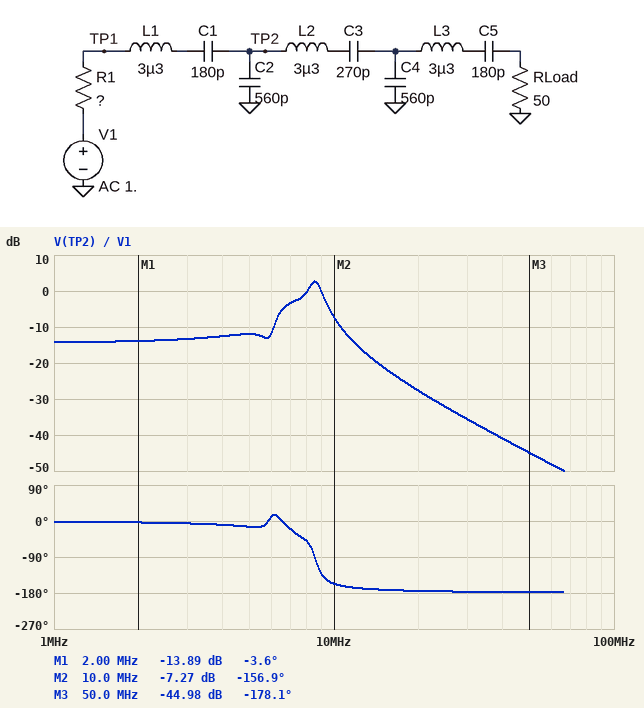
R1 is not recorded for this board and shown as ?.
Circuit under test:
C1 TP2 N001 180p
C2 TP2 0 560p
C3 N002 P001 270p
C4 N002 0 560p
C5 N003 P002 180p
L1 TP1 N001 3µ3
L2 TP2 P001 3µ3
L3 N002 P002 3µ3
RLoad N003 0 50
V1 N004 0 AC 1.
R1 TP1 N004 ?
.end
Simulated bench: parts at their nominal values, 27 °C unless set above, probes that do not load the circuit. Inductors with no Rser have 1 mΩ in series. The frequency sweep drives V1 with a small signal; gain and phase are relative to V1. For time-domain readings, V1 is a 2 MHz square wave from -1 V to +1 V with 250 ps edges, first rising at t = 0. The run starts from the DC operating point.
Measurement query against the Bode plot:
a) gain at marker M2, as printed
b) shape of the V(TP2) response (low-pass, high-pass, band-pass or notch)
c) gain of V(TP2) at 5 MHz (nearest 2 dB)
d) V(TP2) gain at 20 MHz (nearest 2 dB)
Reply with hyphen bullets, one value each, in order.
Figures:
- -7.27 dB
- low-pass
- -12 dB
- -28 dB
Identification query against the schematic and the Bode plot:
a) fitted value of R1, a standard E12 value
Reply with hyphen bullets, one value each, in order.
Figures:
- 33 Ω
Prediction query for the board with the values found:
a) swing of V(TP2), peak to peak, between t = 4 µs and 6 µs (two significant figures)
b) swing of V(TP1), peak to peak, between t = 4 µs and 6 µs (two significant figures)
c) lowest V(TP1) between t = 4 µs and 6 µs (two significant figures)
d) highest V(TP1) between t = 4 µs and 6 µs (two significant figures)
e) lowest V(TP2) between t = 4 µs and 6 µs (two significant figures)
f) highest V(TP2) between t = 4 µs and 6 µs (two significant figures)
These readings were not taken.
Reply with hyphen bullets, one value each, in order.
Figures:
- 740 mV
- 2.6 V
- -1.3 V
- 1.3 V
- -180 mV
- 560 mV
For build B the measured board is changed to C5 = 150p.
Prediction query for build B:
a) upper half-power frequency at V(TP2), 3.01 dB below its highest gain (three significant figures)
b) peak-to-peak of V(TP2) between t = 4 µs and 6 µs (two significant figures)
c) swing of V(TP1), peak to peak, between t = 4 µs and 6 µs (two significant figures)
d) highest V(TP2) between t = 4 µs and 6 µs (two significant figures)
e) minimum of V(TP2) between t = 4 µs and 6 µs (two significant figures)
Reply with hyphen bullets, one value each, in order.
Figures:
- 9.13 MHz
- 680 mV
- 2.6 V
- 530 mV
- -150 mV
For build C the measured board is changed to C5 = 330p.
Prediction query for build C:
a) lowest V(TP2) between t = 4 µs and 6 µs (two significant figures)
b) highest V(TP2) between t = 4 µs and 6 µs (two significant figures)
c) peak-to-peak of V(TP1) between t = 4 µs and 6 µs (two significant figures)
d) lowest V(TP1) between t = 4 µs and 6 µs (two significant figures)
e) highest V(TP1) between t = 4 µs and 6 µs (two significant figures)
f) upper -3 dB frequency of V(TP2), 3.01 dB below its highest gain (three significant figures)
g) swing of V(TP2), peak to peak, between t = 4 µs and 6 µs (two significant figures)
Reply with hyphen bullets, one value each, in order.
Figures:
- -240 mV
- 620 mV
- 2.5 V
- -1.2 V
- 1.2 V
- 8.83 MHz
- 850 mV
